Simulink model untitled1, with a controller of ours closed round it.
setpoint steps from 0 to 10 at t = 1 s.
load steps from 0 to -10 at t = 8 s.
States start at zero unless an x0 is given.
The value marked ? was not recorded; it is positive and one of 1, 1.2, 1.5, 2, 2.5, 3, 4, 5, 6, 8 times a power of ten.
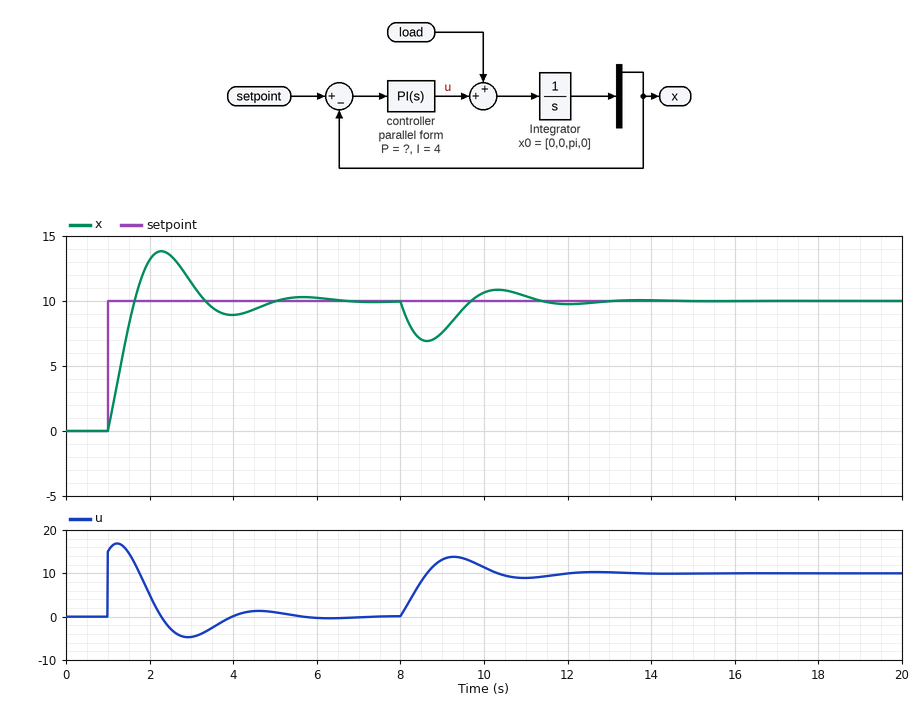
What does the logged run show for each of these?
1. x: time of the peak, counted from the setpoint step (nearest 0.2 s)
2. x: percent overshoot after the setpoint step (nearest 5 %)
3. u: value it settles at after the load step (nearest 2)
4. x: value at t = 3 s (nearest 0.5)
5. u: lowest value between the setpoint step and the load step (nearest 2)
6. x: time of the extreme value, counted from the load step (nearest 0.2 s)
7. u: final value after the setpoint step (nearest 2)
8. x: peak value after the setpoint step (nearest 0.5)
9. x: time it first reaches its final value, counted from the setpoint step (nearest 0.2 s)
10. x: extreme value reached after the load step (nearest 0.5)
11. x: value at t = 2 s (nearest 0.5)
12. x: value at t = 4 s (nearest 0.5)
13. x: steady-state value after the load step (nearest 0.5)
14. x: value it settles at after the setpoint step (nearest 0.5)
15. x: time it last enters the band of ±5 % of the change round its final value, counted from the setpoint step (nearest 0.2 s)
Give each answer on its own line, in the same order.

1.2 s
40 %
10
11.5
-4
0.6 s
0
14.0
0.6 s
7.0
13.0
9.0
10.0
10.0
3.6 s
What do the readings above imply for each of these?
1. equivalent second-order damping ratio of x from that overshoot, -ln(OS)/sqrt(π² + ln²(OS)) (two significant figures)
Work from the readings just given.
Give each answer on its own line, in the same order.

0.28
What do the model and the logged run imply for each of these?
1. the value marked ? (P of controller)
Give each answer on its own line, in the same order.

1.5
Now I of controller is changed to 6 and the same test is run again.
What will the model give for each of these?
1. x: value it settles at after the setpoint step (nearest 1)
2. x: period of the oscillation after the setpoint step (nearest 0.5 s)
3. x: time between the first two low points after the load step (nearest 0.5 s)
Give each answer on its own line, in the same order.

10
2.5 s
2.5 s
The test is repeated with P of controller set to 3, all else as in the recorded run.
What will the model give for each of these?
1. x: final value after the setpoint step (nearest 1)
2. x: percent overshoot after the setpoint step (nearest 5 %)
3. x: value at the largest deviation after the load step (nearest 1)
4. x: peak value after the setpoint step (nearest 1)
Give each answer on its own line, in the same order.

10
20 %
8
12
